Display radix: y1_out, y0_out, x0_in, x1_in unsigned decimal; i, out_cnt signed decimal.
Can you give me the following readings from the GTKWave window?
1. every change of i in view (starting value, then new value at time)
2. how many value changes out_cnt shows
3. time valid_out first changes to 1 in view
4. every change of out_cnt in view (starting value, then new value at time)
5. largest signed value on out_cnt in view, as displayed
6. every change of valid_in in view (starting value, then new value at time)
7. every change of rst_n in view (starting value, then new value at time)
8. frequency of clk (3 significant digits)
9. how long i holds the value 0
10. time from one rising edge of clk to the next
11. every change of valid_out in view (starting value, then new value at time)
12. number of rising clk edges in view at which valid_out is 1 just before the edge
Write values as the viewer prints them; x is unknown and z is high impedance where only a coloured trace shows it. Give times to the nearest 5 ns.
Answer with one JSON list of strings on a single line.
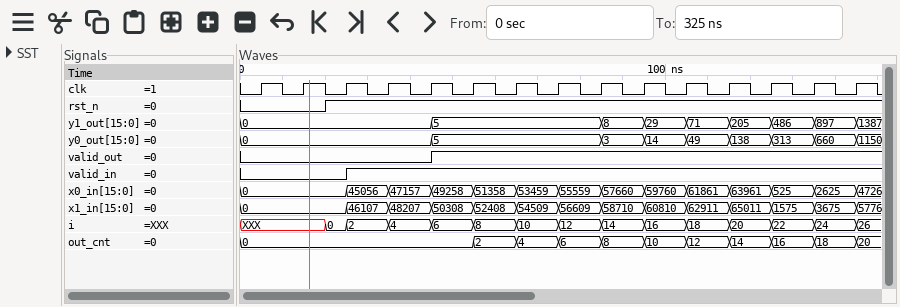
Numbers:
["XXX, 0 at 20 ns, 2 at 25 ns, 4 at 35 ns, 6 at 45 ns, 8 at 55 ns, 10 at 65 ns, 12 at 75 ns, 14 at 85 ns, 16 at 95 ns, 18 at 105 ns, 20 at 115 ns, 22 at 125 ns, 24 at 135 ns, 26 at 145 ns", "10", "45 ns", "0, 2 at 55 ns, 4 at 65 ns, 6 at 75 ns, 8 at 85 ns, 10 at 95 ns, 12 at 105 ns, 14 at 115 ns, 16 at 125 ns, 18 at 135 ns, 20 at 145 ns", "20", "0, 1 at 25 ns", "0, 1 at 20 ns", "100 MHz", "5 ns", "10 ns", "0, 1 at 45 ns", "10"]
